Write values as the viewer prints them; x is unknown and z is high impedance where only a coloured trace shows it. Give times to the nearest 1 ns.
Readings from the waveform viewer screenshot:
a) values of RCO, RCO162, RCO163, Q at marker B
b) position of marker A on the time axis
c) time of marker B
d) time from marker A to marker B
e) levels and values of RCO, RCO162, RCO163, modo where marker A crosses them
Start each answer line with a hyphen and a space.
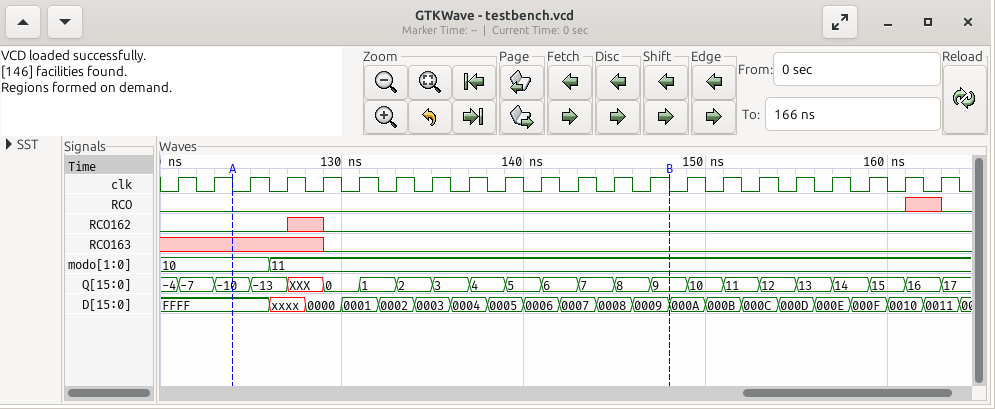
- RCO=0, RCO162=0, RCO163=0, Q=9
- 124 ns
- 148 ns
- 24 ns
- RCO=0, RCO162=0, RCO163=x, modo=10
